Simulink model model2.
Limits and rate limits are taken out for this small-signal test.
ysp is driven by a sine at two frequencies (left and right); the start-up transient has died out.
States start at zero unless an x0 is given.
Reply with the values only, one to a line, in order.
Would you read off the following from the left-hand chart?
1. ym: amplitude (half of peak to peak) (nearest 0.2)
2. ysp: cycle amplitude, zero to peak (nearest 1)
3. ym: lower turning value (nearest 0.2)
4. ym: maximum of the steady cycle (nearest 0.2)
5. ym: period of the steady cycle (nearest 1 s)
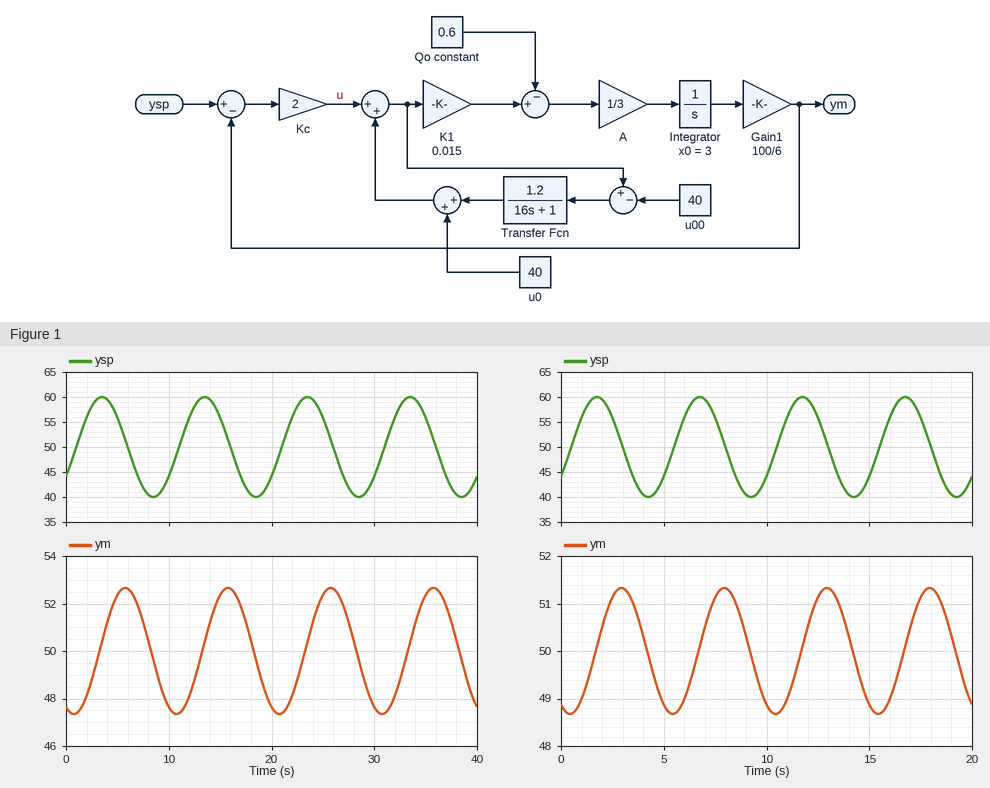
2.6
10
47.4
52.6
10 s
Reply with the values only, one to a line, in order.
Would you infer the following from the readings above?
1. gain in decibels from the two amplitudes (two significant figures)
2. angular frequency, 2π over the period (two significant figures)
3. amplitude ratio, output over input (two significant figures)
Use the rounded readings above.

-12 dB
0.63 rad/s
0.26
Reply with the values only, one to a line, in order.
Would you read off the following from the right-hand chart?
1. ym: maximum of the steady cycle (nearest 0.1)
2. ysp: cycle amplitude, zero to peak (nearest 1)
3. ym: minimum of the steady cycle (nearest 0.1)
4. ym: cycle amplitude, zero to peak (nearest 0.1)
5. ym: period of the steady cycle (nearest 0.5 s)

51.3
10
48.7
1.3
5.0 s
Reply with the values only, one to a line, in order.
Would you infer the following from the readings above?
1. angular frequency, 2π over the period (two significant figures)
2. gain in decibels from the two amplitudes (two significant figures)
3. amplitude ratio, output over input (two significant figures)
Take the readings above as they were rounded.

1.3 rad/s
-18 dB
0.13
